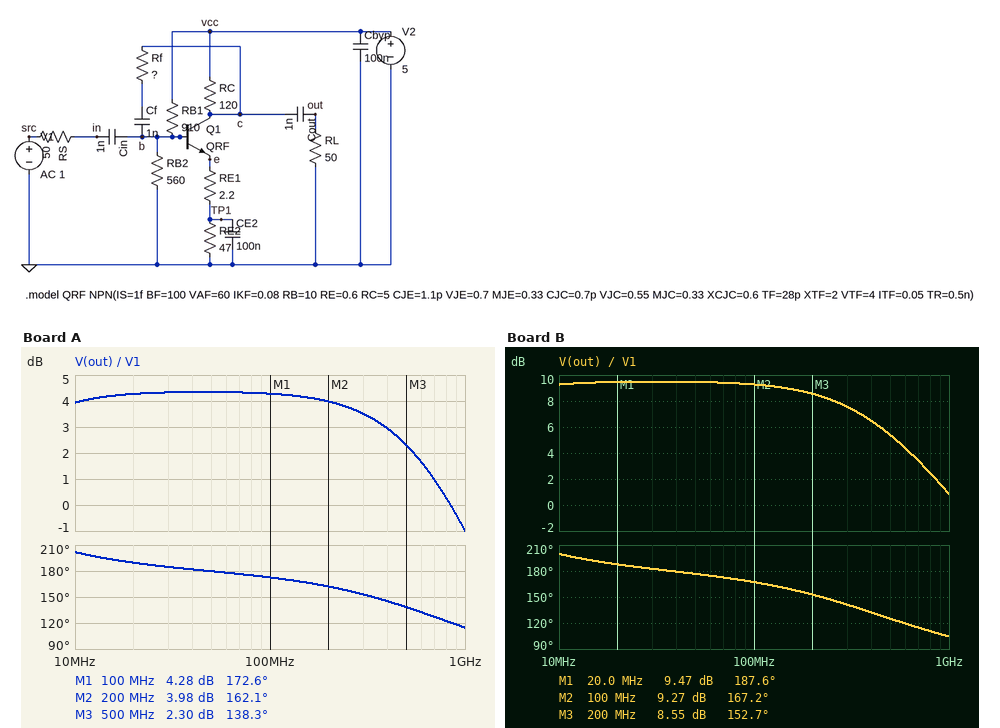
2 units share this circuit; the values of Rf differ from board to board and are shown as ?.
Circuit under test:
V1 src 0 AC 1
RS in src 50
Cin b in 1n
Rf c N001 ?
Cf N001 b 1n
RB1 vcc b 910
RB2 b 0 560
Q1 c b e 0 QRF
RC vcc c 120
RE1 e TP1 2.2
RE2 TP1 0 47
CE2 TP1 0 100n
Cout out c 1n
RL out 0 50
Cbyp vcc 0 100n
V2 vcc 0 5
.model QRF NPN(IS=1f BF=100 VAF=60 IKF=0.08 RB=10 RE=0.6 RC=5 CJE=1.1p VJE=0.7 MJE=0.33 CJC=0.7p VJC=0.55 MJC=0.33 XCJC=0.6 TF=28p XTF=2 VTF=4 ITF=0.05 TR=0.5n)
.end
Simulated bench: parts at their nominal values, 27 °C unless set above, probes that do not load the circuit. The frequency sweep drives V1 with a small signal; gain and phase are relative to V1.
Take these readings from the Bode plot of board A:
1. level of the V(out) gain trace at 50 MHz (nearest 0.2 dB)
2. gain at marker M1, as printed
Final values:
4.4 dB
4.28 dB
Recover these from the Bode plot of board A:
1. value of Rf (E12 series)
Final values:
150 Ω
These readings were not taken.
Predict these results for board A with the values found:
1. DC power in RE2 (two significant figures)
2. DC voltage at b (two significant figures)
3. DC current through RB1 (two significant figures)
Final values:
20 mW
1.8 V
3.5 mA
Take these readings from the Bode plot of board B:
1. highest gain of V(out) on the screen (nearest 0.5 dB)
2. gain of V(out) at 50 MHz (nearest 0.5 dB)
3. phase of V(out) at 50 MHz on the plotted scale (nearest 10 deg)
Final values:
9.5 dB
9.5 dB
180 deg
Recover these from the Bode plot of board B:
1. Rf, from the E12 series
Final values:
390 Ω
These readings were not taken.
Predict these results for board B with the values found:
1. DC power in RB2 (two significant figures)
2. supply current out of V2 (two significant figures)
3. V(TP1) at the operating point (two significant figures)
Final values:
5.9 mW
24 mA
960 mV
